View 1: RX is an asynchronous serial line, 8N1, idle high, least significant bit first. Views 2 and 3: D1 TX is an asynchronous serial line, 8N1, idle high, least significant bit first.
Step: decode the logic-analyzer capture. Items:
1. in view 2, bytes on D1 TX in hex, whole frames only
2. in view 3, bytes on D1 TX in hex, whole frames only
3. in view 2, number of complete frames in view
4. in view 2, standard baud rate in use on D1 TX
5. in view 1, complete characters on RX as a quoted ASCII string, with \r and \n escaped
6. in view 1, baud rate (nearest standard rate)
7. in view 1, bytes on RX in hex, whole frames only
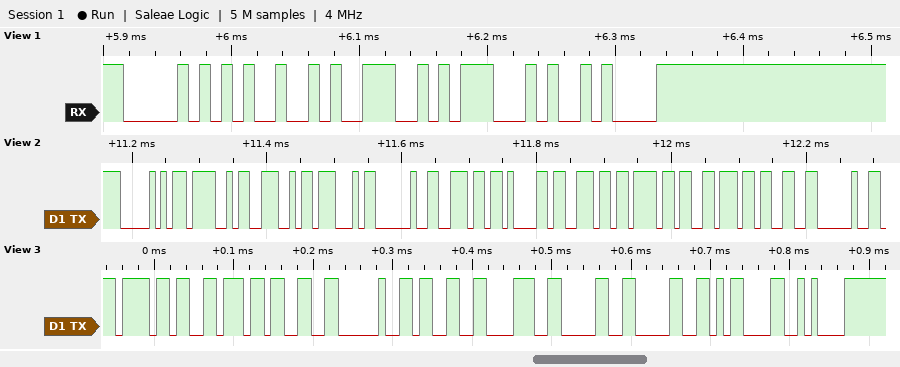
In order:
50 4F 4E 47 20 6E 61 6E 6F 76 33 20
6F 76 33 20 33 38 30 30 0D 0A
12
115200 baud
"PING\n"
115200 baud
50 49 4E 47 0A
